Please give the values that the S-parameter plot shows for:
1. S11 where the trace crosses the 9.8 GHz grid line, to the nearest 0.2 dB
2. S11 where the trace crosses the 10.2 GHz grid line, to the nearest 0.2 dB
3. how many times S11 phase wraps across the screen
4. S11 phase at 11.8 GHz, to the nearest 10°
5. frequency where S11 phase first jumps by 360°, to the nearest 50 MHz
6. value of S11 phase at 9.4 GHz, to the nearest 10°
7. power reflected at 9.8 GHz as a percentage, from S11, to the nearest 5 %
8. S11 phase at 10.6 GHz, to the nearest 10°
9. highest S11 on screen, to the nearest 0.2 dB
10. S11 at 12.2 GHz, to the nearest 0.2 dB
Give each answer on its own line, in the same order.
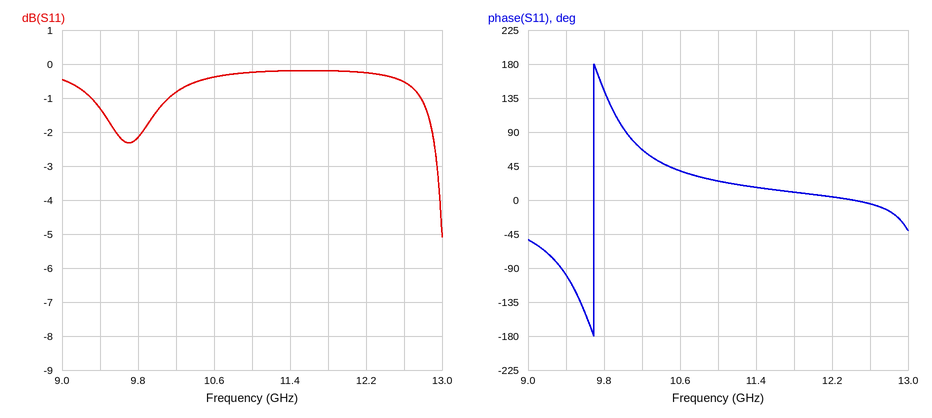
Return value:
-2.2 dB
-0.8 dB
1
10°
9.70 GHz
-100°
60 %
40°
-0.2 dB
-0.2 dB
